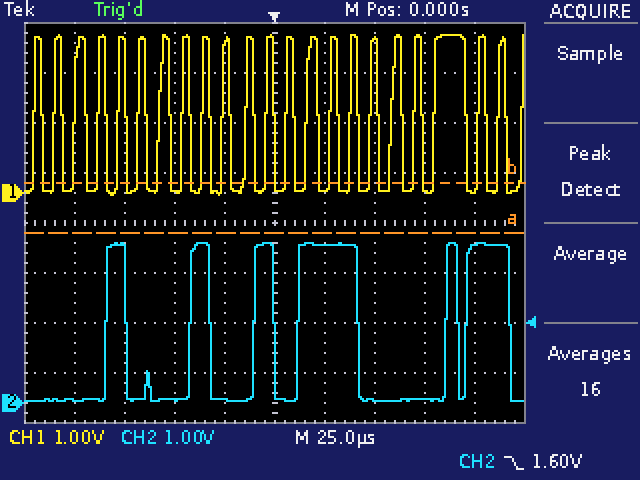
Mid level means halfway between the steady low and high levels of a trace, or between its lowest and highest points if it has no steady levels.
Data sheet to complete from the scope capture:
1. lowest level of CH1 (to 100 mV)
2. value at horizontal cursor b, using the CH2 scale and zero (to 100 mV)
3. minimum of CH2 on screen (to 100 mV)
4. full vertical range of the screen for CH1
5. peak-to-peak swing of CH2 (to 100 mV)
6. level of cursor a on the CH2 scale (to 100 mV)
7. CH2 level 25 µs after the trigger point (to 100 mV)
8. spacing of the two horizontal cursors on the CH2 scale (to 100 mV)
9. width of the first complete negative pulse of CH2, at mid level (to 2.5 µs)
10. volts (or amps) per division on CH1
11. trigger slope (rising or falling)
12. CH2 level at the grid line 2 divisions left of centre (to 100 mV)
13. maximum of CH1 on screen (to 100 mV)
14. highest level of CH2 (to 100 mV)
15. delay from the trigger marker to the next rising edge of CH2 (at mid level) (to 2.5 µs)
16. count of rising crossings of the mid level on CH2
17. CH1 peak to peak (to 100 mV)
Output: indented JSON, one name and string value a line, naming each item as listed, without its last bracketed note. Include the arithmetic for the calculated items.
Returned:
{
  "lowest level of CH1": "0.0 V",
  "value at horizontal cursor b, using the CH2 scale and zero": "4.4 V",
  "minimum of CH2 on screen": "0.0 V",
  "full vertical range of the screen for CH1": "8 V",
  "peak-to-peak swing of CH2": "3.2 V − (0.0 V) = 3.2 V",
  "level of cursor a on the CH2 scale": "3.4 V",
  "CH2 level 25 µs after the trigger point": "3.2 V",
  "spacing of the two horizontal cursors on the CH2 scale": "1.0 V",
  "width of the first complete negative pulse of CH2, at mid level": "32.5 µs",
  "volts (or amps) per division on CH1": "1 V",
  "trigger slope": "falling",
  "CH2 level at the grid line 2 divisions left of centre": "100 mV",
  "maximum of CH1 on screen": "3.2 V",
  "highest level of CH2": "3.2 V",
  "delay from the trigger marker to the next rising edge of CH2 (at mid level)": "12.5 µs",
  "count of rising crossings of the mid level on CH2": "6",
  "CH1 peak to peak": "3.2 V − (0.0 V) = 3.2 V"
}
